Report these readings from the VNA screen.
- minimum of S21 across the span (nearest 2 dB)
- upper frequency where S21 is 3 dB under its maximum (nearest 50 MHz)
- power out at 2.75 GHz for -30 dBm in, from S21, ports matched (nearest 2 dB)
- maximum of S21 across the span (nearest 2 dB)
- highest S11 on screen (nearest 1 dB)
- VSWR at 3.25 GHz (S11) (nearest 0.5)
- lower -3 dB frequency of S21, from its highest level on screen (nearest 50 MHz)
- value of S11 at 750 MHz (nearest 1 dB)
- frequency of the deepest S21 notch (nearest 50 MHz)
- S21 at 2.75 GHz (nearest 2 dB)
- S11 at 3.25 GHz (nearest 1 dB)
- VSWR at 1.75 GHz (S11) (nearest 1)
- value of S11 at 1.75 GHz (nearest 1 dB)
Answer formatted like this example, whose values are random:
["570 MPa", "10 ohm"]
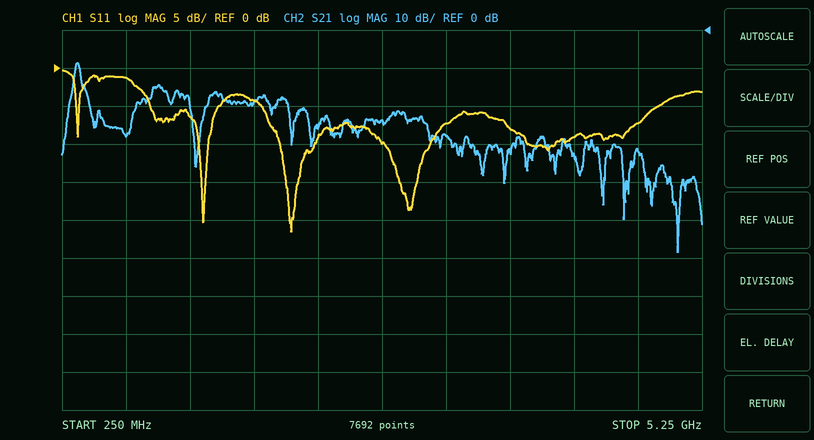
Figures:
["-58 dB", "400 MHz", "-54 dBm", "-8 dB", "0 dB", "2.5", "350 MHz", "-1 dB", "5.05 GHz", "-24 dB", "-7 dB", "4", "-4 dB"]
